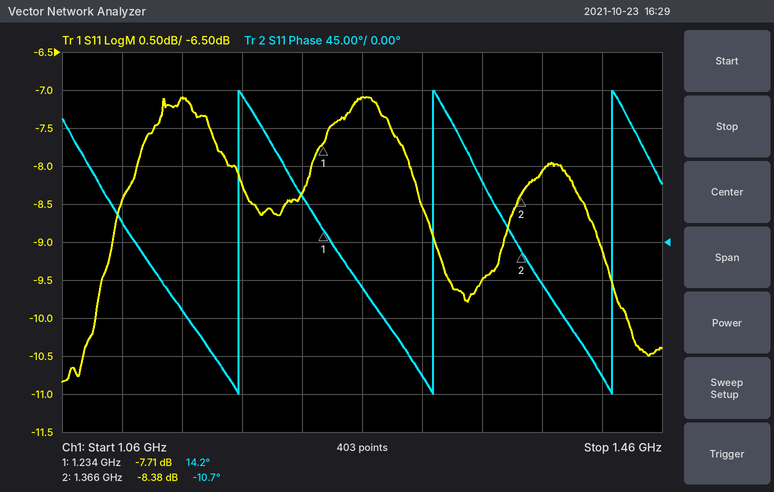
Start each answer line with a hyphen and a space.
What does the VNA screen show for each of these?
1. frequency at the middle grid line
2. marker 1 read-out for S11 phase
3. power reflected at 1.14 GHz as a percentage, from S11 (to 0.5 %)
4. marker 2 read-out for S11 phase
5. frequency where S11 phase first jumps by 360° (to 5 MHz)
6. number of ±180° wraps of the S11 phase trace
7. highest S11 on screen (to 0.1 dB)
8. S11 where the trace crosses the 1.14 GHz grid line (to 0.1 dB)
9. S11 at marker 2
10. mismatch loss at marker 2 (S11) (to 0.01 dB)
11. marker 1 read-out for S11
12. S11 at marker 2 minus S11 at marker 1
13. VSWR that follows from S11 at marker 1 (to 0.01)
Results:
- 1.26 GHz
- 14.2°
- 19.5 %
- -10.7°
- 1.180 GHz
- 3
- -7.1 dB
- -7.1 dB
- -8.38 dB
- 0.68 dB
- -7.71 dB
- -0.67 dB
- 2.40
